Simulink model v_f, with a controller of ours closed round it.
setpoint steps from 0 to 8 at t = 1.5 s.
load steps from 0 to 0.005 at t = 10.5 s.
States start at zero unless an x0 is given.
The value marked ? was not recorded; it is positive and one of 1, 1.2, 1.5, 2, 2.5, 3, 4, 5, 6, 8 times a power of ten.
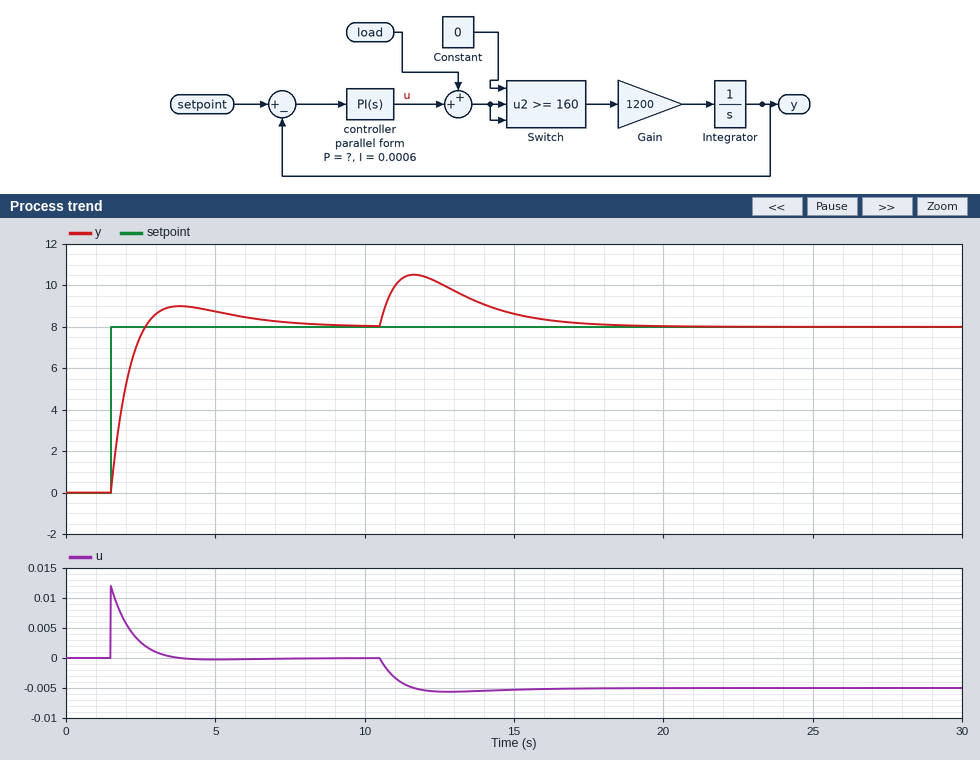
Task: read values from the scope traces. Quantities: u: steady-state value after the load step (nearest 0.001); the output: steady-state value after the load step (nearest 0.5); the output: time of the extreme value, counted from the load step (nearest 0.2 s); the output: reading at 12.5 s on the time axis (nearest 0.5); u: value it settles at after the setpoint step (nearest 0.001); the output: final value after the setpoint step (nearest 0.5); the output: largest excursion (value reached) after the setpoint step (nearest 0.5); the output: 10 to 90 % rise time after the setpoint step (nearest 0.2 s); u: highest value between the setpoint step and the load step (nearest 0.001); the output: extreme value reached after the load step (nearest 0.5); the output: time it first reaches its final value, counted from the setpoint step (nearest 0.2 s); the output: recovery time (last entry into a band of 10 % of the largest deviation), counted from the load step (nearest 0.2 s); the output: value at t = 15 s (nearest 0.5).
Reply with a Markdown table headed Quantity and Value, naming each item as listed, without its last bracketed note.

| Quantity | Value |
|---|---|
| u: steady-state value after the load step | -0.005 |
| the output: steady-state value after the load step | 8.0 |
| the output: time of the extreme value, counted from the load step | 1.2 s |
| the output: reading at 12.5 s on the time axis | 10.0 |
| u: value it settles at after the setpoint step | 0.000 |
| the output: final value after the setpoint step | 8.0 |
| the output: largest excursion (value reached) after the setpoint step | 9.0 |
| the output: 10 to 90 % rise time after the setpoint step | 0.8 s |
| u: highest value between the setpoint step and the load step | 0.012 |
| the output: extreme value reached after the load step | 10.5 |
| the output: time it first reaches its final value, counted from the setpoint step | 1.2 s |
| the output: recovery time (last entry into a band of 10 % of the largest deviation), counted from the load step | 6.2 s |
| the output: value at t = 15 s | 8.5 |
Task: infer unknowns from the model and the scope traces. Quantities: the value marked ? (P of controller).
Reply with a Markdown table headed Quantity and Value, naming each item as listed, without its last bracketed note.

| Quantity | Value |
|---|---|
| the value marked ? | 0.0015 |
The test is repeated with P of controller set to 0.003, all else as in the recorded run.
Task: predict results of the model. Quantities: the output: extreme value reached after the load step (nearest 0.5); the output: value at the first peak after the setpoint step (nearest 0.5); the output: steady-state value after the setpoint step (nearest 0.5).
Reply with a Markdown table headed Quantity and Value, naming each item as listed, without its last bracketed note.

| Quantity | Value |
|---|---|
| the output: extreme value reached after the load step | 9.5 |
| the output: value at the first peak after the setpoint step | 8.5 |
| the output: steady-state value after the setpoint step | 8.0 |
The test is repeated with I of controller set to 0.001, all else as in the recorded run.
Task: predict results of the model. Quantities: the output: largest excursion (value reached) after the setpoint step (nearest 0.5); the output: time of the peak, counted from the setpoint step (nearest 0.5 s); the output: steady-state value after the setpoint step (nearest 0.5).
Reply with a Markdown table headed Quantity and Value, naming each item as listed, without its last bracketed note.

| Quantity | Value |
|---|---|
| the output: largest excursion (value reached) after the setpoint step | 9.5 |
| the output: time of the peak, counted from the setpoint step | 2.0 s |
| the output: steady-state value after the setpoint step | 8.0 |
